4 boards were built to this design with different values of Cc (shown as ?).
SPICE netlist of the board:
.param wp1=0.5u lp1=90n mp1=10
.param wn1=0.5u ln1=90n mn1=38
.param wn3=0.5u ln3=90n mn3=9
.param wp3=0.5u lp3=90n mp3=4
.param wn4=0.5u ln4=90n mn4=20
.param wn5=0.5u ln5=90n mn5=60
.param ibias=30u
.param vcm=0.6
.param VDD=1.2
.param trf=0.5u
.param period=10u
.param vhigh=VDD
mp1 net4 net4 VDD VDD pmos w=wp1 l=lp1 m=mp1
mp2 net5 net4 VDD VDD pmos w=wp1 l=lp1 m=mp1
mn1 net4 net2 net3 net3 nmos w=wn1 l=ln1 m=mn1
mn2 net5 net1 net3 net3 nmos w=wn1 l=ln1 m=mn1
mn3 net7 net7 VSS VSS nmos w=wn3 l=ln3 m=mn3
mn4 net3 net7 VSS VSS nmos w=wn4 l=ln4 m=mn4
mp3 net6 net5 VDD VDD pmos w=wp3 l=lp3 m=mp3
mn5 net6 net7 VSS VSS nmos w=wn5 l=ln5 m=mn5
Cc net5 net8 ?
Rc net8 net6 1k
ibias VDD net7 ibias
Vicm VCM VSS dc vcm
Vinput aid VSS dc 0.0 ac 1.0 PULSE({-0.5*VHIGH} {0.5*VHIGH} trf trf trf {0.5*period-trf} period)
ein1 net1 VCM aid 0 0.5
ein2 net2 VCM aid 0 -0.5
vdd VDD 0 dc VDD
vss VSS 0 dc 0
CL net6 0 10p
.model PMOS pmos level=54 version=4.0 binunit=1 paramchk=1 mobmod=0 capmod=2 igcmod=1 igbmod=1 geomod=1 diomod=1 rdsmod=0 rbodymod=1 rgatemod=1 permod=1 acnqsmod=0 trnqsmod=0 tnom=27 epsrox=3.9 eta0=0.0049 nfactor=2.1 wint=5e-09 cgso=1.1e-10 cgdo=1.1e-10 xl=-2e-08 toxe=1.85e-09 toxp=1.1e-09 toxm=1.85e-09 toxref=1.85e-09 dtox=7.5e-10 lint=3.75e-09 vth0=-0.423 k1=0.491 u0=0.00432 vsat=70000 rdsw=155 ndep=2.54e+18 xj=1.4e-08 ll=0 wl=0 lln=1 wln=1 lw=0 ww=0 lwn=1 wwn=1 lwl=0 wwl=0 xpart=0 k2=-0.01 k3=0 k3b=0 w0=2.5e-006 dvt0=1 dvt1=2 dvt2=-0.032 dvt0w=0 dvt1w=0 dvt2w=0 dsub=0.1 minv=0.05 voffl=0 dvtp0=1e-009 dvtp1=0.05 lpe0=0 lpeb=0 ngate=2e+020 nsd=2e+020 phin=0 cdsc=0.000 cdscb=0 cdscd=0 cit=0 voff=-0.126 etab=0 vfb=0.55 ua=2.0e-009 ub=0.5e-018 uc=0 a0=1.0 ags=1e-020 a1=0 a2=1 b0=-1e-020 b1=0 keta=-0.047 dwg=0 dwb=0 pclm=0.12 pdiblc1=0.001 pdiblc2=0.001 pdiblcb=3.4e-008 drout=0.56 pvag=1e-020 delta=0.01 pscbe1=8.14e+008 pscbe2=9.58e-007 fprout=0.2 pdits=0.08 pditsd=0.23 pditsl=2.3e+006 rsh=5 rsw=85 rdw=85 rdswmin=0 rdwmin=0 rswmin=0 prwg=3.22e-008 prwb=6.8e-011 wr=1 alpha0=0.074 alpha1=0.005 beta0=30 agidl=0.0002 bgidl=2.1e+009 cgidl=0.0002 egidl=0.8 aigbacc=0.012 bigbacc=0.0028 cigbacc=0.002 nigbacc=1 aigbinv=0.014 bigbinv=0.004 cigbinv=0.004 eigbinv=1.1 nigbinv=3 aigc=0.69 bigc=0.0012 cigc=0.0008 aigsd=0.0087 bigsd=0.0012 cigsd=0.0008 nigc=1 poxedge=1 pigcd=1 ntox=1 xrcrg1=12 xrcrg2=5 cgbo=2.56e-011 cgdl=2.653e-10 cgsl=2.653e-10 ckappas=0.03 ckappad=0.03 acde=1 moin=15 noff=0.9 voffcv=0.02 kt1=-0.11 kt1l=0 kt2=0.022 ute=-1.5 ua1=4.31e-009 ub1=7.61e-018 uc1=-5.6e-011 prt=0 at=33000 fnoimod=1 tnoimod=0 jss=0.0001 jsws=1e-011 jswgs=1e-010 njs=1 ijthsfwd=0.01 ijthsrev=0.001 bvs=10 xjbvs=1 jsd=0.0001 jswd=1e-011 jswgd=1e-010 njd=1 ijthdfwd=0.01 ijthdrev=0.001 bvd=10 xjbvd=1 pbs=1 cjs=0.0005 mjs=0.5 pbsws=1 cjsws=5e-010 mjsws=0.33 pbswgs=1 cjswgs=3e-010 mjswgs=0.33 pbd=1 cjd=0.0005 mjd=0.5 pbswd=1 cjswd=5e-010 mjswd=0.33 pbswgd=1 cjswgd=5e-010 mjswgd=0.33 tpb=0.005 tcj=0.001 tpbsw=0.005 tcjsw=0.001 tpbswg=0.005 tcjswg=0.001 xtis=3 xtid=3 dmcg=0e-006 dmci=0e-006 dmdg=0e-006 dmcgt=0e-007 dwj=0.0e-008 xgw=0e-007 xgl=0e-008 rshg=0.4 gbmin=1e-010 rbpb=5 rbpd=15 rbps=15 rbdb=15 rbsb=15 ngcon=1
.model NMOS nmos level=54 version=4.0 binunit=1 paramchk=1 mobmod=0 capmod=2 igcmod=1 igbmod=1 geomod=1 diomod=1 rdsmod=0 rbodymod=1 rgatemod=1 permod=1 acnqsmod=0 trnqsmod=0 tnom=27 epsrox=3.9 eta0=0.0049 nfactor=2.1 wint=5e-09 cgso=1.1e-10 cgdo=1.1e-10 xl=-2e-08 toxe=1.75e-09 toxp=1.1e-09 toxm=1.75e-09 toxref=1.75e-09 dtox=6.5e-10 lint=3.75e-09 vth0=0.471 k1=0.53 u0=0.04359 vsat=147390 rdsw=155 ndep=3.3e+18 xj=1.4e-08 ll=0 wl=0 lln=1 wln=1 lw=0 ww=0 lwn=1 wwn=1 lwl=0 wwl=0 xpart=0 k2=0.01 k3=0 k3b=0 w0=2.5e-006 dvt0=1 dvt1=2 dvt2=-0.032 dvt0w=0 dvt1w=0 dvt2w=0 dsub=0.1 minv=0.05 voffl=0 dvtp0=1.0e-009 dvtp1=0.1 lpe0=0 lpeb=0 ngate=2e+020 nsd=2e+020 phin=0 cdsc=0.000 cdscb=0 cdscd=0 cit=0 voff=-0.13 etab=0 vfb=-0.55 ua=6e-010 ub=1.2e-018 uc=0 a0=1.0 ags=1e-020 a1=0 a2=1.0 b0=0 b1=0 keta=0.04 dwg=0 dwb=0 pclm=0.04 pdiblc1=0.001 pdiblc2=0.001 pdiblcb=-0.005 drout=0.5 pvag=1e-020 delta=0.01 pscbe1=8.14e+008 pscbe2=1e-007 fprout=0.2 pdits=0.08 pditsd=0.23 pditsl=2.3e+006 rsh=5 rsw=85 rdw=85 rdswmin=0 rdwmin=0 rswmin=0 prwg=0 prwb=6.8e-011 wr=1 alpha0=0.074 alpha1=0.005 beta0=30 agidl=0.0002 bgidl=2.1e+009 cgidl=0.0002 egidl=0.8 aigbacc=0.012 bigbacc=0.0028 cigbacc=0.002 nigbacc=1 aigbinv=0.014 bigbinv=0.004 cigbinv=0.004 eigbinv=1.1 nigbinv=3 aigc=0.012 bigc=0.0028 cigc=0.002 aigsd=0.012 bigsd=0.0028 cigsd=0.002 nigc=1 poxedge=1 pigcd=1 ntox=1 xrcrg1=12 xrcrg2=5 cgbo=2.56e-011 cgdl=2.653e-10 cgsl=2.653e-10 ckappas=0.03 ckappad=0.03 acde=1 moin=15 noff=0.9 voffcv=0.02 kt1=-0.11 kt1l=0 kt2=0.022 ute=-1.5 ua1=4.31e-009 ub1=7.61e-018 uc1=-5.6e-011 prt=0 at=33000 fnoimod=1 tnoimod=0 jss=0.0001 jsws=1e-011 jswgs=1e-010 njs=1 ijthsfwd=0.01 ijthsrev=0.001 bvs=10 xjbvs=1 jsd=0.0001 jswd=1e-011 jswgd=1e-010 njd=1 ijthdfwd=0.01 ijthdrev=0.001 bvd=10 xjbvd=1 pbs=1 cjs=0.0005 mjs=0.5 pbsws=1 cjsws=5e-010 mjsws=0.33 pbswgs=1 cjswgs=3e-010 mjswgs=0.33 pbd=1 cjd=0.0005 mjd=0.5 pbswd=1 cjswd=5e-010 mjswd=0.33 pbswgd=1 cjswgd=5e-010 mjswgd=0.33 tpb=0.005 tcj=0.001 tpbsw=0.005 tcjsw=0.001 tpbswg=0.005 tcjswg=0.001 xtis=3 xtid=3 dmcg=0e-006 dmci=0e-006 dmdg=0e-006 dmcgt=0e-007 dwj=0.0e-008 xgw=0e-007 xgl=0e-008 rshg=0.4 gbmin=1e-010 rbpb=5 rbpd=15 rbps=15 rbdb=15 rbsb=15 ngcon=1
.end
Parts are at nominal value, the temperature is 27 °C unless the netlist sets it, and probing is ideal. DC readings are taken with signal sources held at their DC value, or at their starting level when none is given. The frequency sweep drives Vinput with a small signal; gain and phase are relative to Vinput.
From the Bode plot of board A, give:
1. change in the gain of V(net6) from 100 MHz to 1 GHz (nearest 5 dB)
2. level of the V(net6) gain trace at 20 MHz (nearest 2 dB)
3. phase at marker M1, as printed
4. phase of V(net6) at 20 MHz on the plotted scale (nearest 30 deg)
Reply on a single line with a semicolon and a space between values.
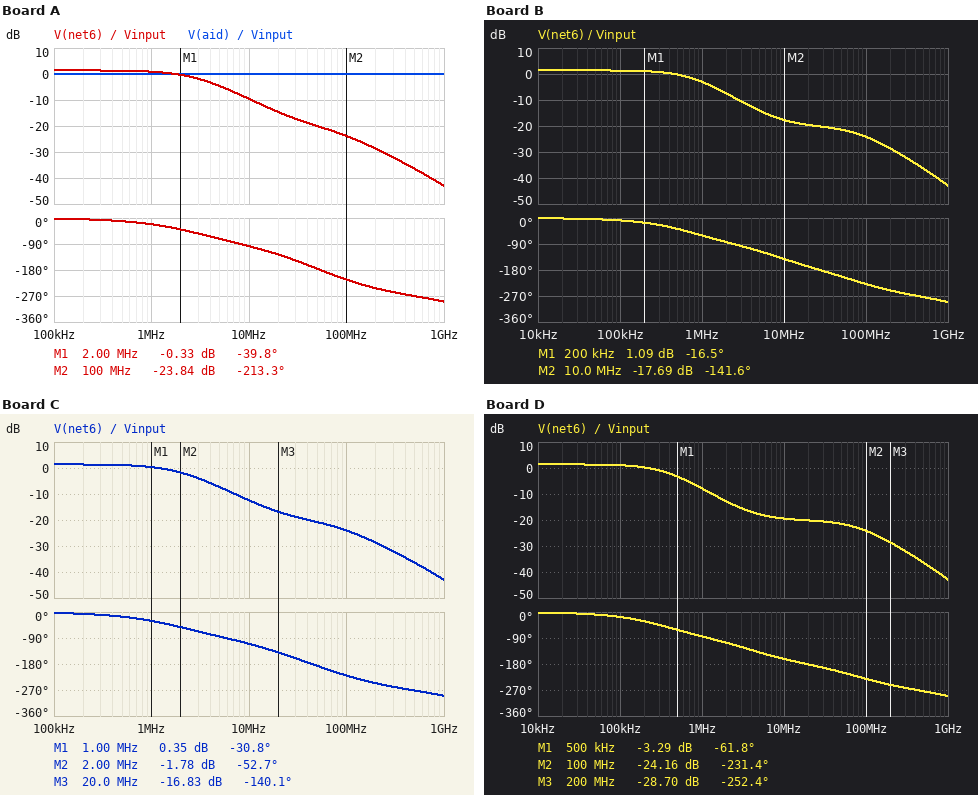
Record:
-20 dB; -14 dB; -39.8 deg; -120 deg
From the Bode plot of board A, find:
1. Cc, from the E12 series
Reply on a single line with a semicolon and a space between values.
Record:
1 pF
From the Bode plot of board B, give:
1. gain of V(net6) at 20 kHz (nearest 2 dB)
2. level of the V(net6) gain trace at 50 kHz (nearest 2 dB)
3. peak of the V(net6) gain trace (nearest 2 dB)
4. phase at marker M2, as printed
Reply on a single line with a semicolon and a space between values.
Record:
2 dB; 2 dB; 2 dB; -141.6 deg
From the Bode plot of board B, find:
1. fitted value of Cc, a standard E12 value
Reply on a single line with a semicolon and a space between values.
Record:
3.9 pF
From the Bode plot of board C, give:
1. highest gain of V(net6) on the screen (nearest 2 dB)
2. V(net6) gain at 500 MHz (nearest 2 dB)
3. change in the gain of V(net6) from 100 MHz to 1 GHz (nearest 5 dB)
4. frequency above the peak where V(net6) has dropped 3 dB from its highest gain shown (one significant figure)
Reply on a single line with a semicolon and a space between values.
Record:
2 dB; -36 dB; -20 dB; 2 MHz
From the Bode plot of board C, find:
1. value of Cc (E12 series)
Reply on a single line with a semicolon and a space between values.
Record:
1.5 pF
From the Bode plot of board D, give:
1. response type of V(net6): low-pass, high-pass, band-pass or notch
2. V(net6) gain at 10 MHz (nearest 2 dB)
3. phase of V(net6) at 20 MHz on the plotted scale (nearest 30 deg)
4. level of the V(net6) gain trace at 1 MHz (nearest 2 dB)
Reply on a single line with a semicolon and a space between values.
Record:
low-pass; -20 dB; -180 deg; -8 dB
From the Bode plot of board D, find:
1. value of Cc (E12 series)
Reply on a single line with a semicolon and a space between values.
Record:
8.2 pF
